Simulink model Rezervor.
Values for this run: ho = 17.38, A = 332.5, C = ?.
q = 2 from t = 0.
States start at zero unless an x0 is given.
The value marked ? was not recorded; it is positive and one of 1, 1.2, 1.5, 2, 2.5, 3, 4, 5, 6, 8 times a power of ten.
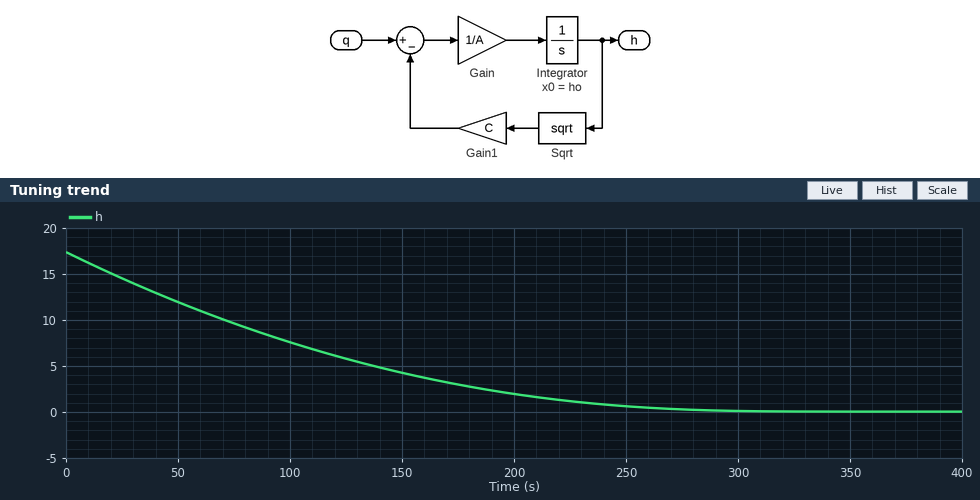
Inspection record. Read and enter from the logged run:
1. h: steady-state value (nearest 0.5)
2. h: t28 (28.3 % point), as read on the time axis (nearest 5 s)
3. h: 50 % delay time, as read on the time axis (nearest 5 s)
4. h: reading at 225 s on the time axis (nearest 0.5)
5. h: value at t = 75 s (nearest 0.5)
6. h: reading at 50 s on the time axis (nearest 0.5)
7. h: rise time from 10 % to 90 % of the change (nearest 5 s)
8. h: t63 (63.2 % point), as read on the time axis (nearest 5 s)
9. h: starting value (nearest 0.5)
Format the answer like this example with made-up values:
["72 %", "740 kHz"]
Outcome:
["0.0", "45 s", "85 s", "1.0", "9.5", "12.0", "190 s", "115 s", "17.5"]
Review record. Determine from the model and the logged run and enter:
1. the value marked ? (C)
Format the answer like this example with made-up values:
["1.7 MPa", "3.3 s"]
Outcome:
["10"]
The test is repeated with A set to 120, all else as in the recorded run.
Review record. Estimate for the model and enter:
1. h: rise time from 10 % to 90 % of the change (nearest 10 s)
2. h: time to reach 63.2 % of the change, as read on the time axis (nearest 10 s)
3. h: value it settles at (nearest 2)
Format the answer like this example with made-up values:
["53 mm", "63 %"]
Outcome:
["70 s", "40 s", "0"]
